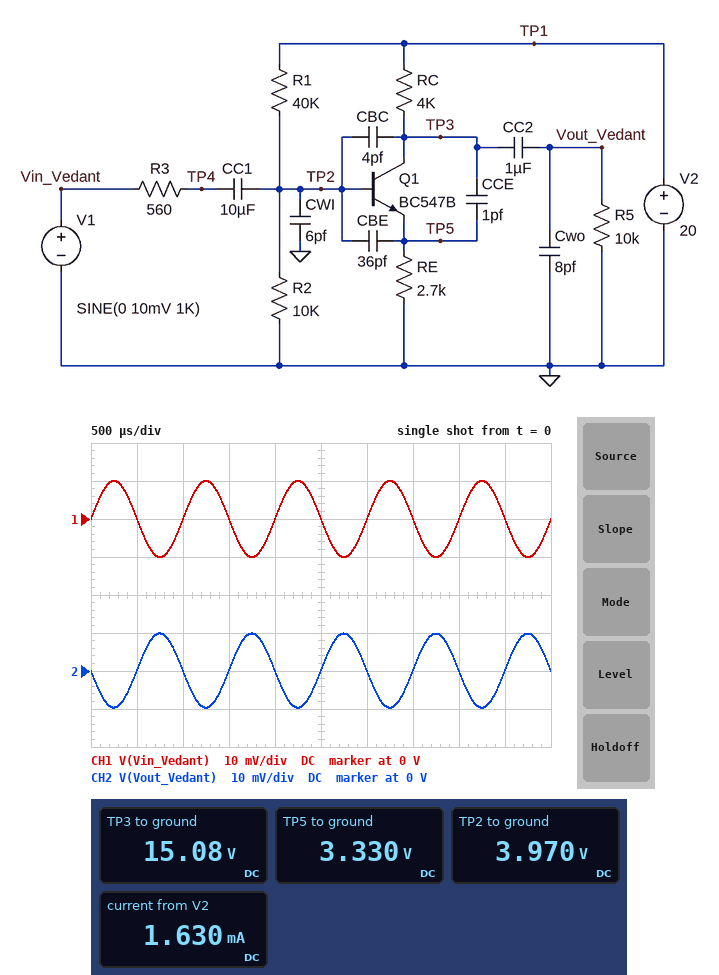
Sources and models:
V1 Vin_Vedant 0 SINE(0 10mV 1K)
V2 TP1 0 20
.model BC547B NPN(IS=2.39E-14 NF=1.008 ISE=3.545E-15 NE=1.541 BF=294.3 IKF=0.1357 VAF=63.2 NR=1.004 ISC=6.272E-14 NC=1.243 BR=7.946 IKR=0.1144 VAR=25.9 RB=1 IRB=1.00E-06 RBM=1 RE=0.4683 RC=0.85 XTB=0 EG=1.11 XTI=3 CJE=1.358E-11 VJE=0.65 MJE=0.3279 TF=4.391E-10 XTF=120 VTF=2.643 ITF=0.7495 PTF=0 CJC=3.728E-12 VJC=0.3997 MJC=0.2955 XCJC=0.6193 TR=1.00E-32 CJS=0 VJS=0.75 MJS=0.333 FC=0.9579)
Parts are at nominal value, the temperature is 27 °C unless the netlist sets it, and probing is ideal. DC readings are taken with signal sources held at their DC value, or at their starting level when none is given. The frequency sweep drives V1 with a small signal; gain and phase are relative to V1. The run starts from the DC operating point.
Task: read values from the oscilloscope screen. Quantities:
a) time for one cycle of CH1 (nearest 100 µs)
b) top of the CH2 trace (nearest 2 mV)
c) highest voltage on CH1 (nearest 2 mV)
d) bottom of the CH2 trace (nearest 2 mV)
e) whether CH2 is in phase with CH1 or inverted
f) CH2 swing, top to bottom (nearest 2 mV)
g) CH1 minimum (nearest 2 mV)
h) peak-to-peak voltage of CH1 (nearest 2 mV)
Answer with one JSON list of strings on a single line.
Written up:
["1.0 ms", "10 mV", "10 mV", "-10 mV", "inverted", "20 mV", "-10 mV", "20 mV"]
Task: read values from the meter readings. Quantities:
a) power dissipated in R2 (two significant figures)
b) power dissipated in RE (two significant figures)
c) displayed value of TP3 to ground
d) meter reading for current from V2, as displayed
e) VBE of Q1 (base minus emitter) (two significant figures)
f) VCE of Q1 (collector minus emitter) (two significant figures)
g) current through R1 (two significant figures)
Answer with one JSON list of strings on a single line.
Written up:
["1.6 mW", "4.1 mW", "15.08 V", "1.630 mA", "640 mV", "12 V", "400 µA"]
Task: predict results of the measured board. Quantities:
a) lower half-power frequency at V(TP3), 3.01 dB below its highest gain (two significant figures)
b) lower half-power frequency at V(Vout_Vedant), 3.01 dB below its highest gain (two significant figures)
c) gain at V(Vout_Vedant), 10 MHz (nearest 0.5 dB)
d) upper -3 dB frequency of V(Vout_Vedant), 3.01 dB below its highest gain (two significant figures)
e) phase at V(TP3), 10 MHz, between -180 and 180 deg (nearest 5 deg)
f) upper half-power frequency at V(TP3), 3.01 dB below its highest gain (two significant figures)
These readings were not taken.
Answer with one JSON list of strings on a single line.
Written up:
["1.6 Hz", "12 Hz", "-6.5 dB", "4.4 MHz", "45 deg", "2.1 MHz"]
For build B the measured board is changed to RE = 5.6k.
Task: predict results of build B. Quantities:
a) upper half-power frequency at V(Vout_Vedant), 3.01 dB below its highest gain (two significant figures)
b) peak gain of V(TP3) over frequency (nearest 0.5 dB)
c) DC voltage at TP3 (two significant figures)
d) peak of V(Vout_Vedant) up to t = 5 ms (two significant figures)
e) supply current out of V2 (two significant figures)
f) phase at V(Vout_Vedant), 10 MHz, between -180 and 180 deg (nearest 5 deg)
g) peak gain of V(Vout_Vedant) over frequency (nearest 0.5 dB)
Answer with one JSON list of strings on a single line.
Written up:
["21 MHz", "-4.5 dB", "18 V", "4.8 mV", "1.0 mA", "30 deg", "-6.5 dB"]
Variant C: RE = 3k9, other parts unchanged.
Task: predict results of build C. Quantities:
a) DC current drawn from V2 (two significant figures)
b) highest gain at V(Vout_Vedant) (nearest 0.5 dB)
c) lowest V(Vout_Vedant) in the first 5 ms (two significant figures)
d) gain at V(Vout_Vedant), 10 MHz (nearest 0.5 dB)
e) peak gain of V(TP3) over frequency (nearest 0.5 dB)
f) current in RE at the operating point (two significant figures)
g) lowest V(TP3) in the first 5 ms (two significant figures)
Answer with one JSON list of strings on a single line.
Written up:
["1.3 mA", "-3.5 dB", "-6.7 mV", "-7.5 dB", "-1.5 dB", "860 µA", "17 V"]
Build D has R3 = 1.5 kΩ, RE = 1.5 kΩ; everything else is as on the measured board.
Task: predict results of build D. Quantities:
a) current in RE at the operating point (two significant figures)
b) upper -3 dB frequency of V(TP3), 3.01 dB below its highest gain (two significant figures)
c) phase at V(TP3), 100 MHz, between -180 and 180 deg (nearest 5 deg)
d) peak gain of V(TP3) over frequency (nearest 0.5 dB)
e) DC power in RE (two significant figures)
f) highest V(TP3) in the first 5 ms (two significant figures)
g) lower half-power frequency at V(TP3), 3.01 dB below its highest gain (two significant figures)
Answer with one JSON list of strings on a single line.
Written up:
["2.2 mA", "1.3 MHz", "-70 deg", "6.0 dB", "7.2 mW", "11 V", "1.4 Hz"]
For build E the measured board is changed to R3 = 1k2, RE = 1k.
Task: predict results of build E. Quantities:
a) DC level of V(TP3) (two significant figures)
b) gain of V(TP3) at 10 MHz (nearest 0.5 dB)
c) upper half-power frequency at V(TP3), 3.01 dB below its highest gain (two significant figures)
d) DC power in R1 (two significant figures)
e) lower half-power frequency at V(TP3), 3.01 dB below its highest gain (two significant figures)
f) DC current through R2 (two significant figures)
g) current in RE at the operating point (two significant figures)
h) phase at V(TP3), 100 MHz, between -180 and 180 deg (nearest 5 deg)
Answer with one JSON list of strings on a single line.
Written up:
["7.1 V", "-4.5 dB", "1.2 MHz", "6.5 mW", "1.5 Hz", "390 µA", "3.2 mA", "-65 deg"]
